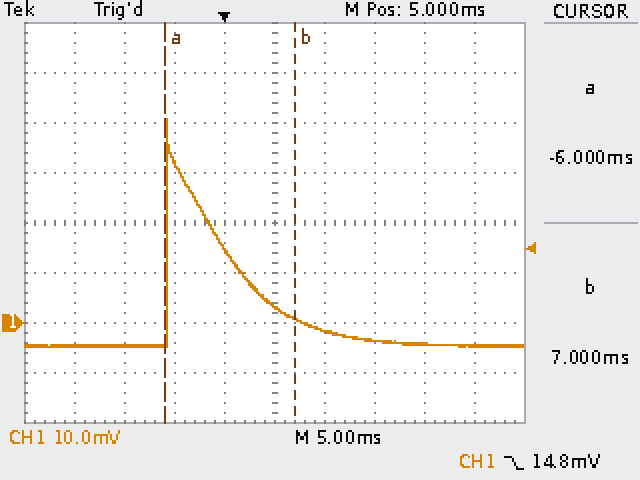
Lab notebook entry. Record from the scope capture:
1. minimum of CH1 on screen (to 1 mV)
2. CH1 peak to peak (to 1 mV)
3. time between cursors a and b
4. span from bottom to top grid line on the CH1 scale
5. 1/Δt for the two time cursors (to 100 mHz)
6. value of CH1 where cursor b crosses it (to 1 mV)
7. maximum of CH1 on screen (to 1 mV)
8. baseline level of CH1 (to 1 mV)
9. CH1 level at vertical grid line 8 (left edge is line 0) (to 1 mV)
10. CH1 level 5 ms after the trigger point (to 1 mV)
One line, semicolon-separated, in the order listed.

-5 mV; 46 mV; 13.0 ms; 80 mV; 76.9 Hz; 1 mV; 41 mV; -5 mV; -4 mV; 3 mV
